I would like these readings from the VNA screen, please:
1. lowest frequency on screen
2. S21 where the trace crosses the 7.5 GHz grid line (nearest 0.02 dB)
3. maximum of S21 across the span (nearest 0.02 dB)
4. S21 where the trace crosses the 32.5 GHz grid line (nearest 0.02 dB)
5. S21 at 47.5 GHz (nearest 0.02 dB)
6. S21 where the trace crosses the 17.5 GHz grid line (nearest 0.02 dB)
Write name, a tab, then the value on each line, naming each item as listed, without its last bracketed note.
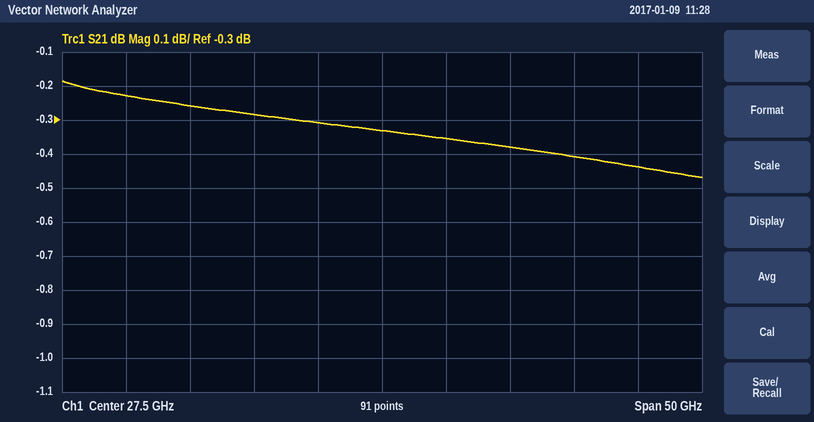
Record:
lowest frequency on screen	2.5 GHz
S21 where the trace crosses the 7.5 GHz grid line	-0.22 dB
maximum of S21 across the span	-0.18 dB
S21 where the trace crosses the 32.5 GHz grid line	-0.36 dB
S21 at 47.5 GHz	-0.44 dB
S21 where the trace crosses the 17.5 GHz grid line	-0.28 dB
